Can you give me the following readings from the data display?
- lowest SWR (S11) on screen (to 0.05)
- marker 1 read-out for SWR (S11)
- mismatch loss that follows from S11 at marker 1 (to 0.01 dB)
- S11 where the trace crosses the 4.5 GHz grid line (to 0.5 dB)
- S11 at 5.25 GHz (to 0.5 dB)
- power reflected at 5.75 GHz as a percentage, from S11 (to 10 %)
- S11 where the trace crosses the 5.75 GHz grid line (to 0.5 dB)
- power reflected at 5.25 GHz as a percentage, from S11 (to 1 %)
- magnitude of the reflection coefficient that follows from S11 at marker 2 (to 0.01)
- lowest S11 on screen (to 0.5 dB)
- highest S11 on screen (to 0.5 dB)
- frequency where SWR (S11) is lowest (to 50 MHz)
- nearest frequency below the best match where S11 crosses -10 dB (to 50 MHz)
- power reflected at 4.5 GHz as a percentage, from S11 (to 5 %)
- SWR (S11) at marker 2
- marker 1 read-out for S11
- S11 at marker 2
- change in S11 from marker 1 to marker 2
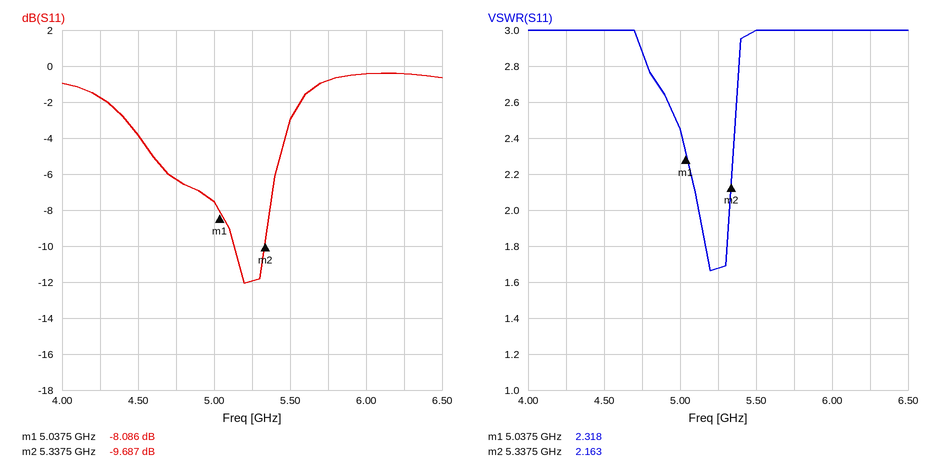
1.65
2.318
0.73 dB
-4.0 dB
-12.0 dB
80 %
-1.0 dB
6 %
0.33
-12.0 dB
-0.5 dB
5.20 GHz
5.15 GHz
40 %
2.163
-8.086 dB
-9.687 dB
-1.601 dB
